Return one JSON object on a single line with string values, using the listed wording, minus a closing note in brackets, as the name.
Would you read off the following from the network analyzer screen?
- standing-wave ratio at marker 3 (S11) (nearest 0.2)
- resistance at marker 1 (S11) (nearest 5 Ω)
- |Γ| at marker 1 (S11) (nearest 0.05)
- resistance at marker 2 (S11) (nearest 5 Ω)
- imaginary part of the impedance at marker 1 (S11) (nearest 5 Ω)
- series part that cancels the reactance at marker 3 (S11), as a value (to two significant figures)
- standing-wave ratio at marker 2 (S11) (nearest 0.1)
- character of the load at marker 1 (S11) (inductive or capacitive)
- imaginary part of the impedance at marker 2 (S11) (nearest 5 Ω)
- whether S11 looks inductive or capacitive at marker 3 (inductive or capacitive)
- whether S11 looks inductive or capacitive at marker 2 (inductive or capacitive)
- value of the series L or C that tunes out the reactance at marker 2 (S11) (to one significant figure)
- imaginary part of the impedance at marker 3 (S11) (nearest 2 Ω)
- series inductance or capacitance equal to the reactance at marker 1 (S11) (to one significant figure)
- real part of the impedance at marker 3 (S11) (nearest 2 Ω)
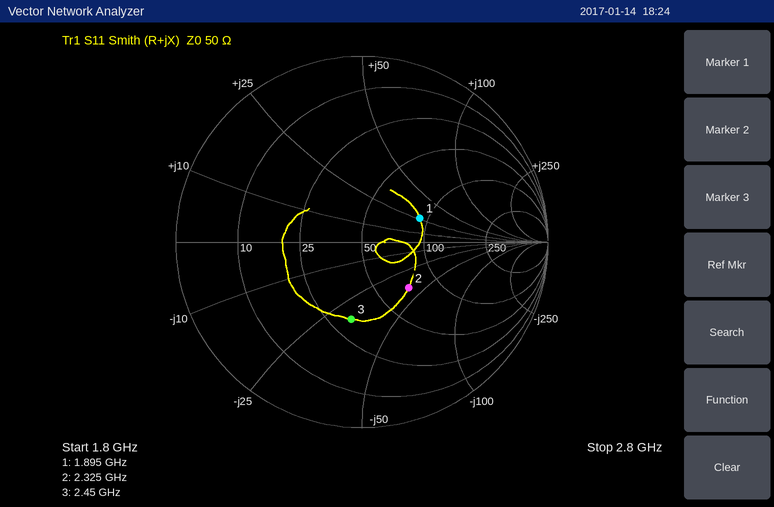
{"standing-wave ratio at marker 3 (S11)": "2.4", "resistance at marker 1 (S11)": "90 Ω", "|Γ| at marker 1 (S11)": "0.35", "resistance at marker 2 (S11)": "70 Ω", "imaginary part of the impedance at marker 1 (S11)": "+25 Ω", "series part that cancels the reactance at marker 3 (S11), as a value": "2.1 nH", "standing-wave ratio at marker 2 (S11)": "2.1", "character of the load at marker 1 (S11)": "inductive", "imaginary part of the impedance at marker 2 (S11)": "-40 Ω", "whether S11 looks inductive or capacitive at marker 3": "capacitive", "whether S11 looks inductive or capacitive at marker 2": "capacitive", "value of the series L or C that tunes out the reactance at marker 2 (S11)": "3 nH", "imaginary part of the impedance at marker 3 (S11)": "-32 Ω", "series inductance or capacitance equal to the reactance at marker 1 (S11)": "2 nH", "real part of the impedance at marker 3 (S11)": "32 Ω"}
